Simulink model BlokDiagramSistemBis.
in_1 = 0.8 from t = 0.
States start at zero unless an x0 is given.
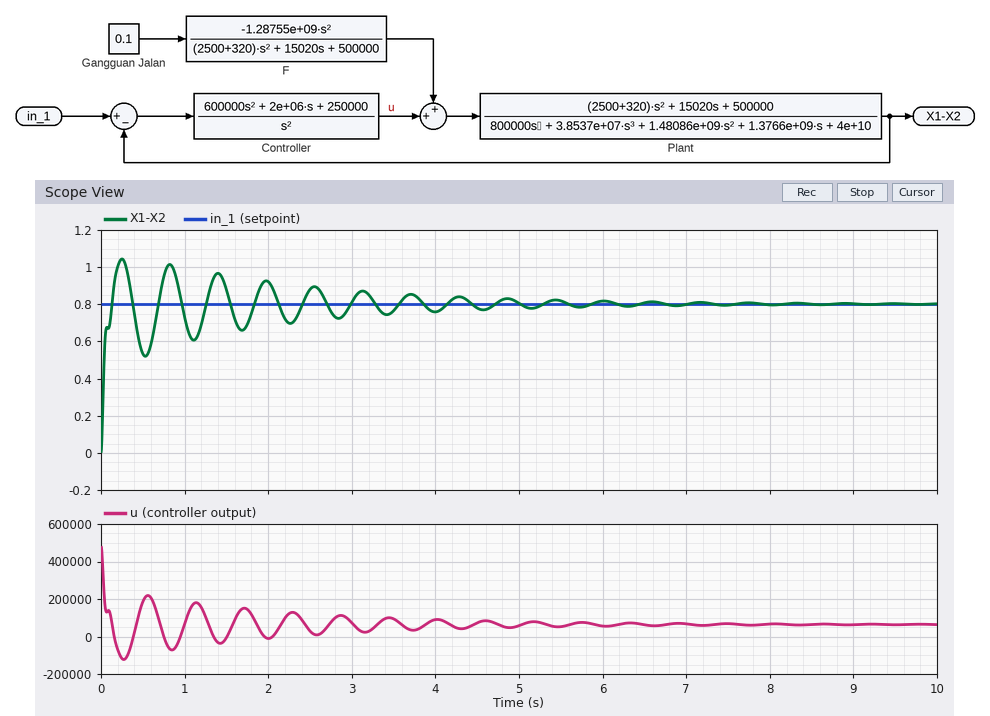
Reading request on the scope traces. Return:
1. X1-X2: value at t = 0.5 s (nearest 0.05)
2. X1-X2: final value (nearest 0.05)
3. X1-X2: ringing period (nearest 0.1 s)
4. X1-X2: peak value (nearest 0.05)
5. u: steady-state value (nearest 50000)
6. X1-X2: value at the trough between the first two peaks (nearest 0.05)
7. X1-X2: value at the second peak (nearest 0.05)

0.55
0.80
0.6 s
1.05
50000
0.50
1.00
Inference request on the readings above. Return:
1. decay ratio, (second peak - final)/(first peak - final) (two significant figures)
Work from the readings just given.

0.80
